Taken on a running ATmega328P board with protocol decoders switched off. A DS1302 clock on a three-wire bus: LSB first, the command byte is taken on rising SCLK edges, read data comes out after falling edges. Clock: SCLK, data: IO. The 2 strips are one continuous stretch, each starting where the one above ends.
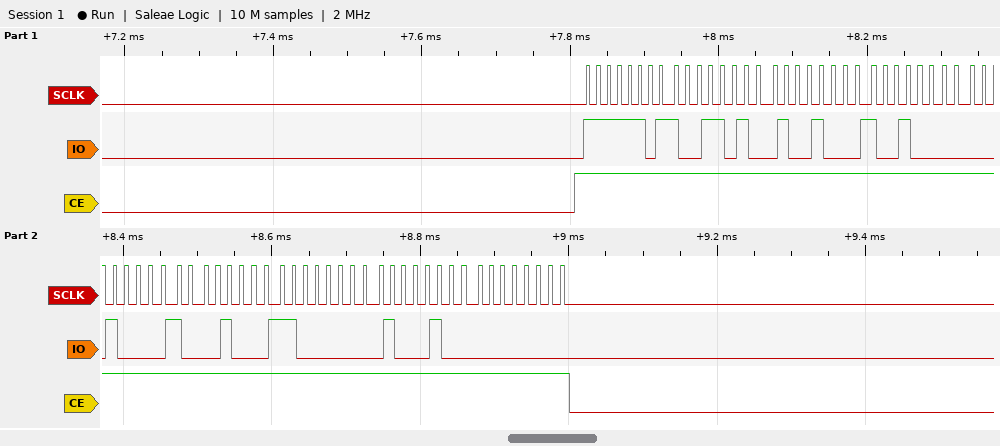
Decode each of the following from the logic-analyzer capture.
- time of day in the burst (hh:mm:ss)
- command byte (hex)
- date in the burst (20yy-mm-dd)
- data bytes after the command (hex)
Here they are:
09:12:59
0xBF
2022-11-08
59 12 09 08 11 03 22 00
